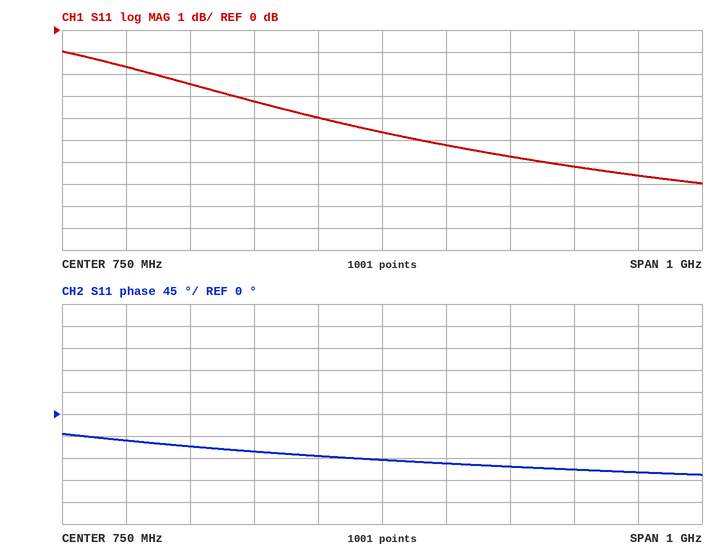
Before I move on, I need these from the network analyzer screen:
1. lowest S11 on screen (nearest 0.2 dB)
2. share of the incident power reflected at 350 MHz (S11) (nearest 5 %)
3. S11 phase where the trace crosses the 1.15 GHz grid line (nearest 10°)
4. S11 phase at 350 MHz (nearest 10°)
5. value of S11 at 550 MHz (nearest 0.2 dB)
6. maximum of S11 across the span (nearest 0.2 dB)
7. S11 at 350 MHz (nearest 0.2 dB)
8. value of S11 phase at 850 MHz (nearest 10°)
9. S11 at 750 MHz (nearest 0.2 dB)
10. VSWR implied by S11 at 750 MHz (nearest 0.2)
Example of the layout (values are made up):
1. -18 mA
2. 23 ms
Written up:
1. -7.0 dB
2. 70 %
3. -120°
4. -50°
5. -3.2 dB
6. -1.0 dB
7. -1.6 dB
8. -100°
9. -4.6 dB
10. 3.8
